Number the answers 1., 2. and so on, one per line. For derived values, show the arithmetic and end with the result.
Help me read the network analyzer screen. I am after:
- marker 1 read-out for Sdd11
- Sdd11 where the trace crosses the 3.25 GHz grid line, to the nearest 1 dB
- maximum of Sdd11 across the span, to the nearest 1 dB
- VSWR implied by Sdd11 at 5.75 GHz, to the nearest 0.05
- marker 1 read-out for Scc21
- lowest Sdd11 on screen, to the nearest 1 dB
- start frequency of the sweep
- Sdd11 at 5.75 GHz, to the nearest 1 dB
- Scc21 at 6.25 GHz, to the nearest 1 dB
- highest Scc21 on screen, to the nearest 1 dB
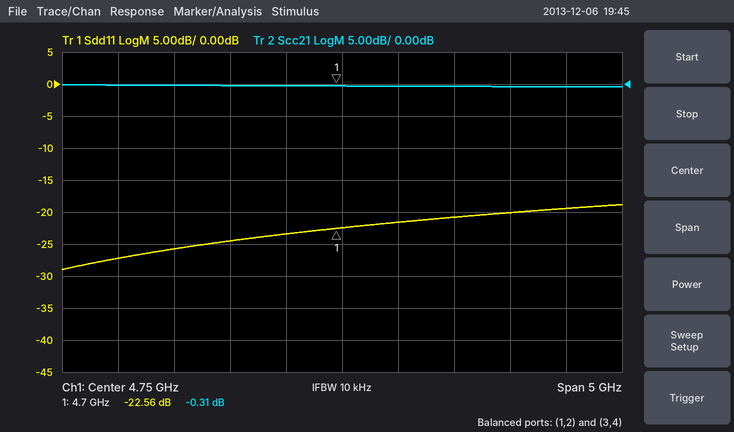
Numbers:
1. -22.56 dB
2. -26 dB
3. -19 dB
4. |Γ| = 10^(-21/20) = 0.0891; VSWR = (1 + 0.0891)/(1 − 0.0891) ≈ 1.20
5. -0.31 dB
6. -29 dB
7. 2.25 GHz
8. -21 dB
9. 0 dB
10. 0 dB
